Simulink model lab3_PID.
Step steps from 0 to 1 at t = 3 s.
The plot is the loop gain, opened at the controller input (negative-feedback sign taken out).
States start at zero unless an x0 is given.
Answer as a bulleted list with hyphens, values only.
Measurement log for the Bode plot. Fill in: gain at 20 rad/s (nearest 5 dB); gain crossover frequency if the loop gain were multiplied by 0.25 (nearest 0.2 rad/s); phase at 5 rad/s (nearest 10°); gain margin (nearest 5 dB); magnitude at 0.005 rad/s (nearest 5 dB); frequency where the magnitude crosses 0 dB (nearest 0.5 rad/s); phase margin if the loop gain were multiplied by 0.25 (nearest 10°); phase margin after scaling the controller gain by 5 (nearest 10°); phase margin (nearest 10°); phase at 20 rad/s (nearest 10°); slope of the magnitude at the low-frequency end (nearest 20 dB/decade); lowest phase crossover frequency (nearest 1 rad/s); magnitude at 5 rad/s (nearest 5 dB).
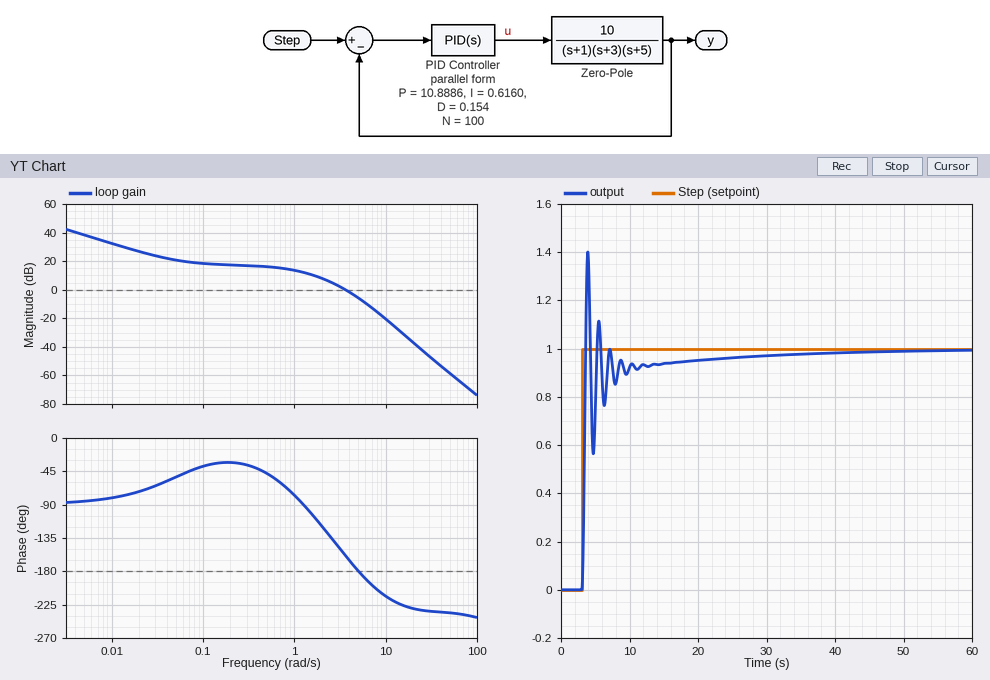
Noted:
- -35 dB
- 1.2 rad/s
- -180°
- 5 dB
- 40 dB
- 3.5 rad/s
- 90°
- -20°
- 20°
- -230°
- -20 dB/decade
- 5 rad/s
- -5 dB
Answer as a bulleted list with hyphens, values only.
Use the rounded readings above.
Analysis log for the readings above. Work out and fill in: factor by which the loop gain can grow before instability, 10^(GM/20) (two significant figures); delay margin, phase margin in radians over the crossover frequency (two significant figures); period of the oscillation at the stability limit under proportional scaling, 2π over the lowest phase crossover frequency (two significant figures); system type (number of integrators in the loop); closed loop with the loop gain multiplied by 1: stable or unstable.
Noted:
- 1.8
- 0.100 s
- 1.3 s
- 1
- stable
